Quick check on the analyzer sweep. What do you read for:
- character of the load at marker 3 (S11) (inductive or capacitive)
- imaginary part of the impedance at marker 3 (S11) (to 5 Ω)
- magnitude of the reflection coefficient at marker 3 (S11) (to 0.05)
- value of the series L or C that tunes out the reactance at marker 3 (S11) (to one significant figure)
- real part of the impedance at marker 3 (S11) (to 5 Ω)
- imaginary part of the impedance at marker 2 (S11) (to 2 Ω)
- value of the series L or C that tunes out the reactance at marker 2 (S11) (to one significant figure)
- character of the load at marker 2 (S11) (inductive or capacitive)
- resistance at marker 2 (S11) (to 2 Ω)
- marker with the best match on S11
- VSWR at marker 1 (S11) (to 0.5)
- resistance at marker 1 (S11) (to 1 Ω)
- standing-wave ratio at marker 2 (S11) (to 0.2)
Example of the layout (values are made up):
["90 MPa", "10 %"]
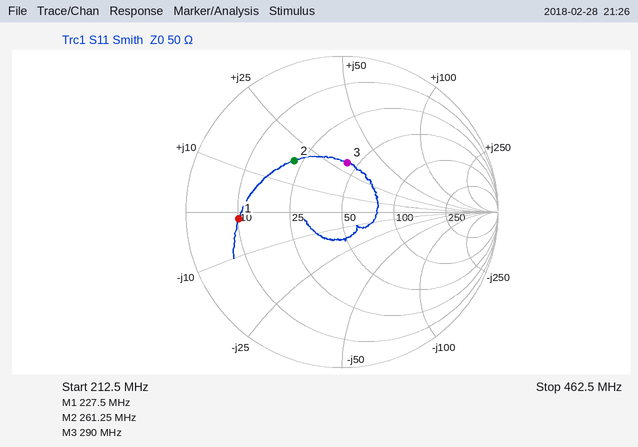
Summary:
["inductive", "+30 Ω", "0.30", "20 pF", "45 Ω", "+18 Ω", "30 pF", "inductive", "22 Ω", "marker 3", "5.0", "10 Ω", "2.6"]
